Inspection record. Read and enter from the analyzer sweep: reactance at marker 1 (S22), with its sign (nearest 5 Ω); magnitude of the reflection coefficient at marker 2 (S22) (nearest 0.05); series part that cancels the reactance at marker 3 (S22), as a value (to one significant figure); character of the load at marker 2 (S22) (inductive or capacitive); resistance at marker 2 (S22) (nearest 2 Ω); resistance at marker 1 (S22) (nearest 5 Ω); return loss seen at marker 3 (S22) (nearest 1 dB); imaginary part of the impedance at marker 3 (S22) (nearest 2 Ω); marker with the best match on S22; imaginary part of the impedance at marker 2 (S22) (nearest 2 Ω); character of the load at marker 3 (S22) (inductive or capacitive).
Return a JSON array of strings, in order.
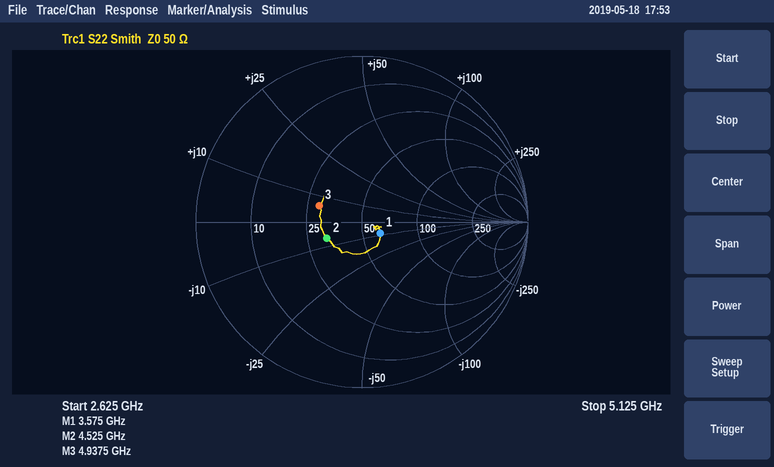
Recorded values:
["-10 Ω", "0.25", "5 pF", "capacitive", "32 Ω", "60 Ω", "11 dB", "+6 Ω", "marker 1", "-6 Ω", "inductive"]
